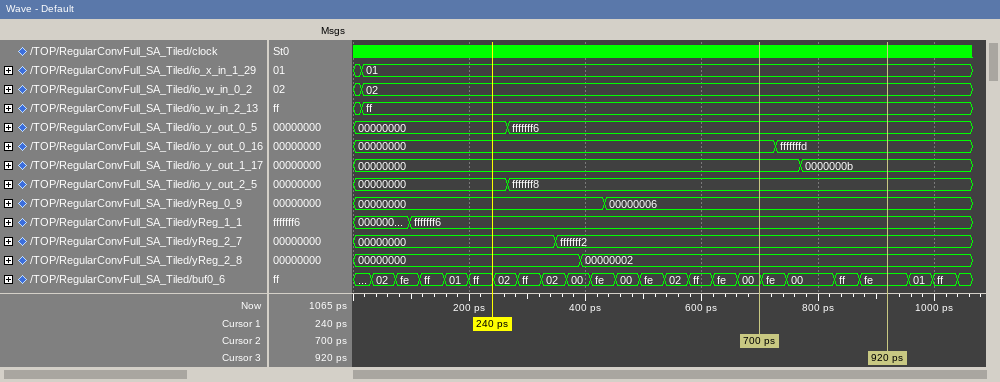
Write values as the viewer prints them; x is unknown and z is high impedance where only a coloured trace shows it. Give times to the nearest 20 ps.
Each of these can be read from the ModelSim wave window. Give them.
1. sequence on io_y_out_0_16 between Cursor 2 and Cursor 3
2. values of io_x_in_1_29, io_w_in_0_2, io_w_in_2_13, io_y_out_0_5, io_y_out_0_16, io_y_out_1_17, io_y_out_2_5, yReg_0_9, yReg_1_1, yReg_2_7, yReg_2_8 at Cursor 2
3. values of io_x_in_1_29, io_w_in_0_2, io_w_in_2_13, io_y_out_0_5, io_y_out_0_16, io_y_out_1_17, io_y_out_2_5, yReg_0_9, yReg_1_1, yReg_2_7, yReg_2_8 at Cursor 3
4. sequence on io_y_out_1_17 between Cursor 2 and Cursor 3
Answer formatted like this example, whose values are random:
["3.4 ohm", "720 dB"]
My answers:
["00000000, fffffffd", "io_x_in_1_29=01, io_w_in_0_2=02, io_w_in_2_13=ff, io_y_out_0_5=fffffff6, io_y_out_0_16=00000000, io_y_out_1_17=00000000, io_y_out_2_5=fffffff8, yReg_0_9=00000006, yReg_1_1=fffffff6, yReg_2_7=fffffff2, yReg_2_8=00000002", "io_x_in_1_29=01, io_w_in_0_2=02, io_w_in_2_13=ff, io_y_out_0_5=fffffff6, io_y_out_0_16=fffffffd, io_y_out_1_17=0000000b, io_y_out_2_5=fffffff8, yReg_0_9=00000006, yReg_1_1=fffffff6, yReg_2_7=fffffff2, yReg_2_8=00000002", "00000000, 0000000b"]
